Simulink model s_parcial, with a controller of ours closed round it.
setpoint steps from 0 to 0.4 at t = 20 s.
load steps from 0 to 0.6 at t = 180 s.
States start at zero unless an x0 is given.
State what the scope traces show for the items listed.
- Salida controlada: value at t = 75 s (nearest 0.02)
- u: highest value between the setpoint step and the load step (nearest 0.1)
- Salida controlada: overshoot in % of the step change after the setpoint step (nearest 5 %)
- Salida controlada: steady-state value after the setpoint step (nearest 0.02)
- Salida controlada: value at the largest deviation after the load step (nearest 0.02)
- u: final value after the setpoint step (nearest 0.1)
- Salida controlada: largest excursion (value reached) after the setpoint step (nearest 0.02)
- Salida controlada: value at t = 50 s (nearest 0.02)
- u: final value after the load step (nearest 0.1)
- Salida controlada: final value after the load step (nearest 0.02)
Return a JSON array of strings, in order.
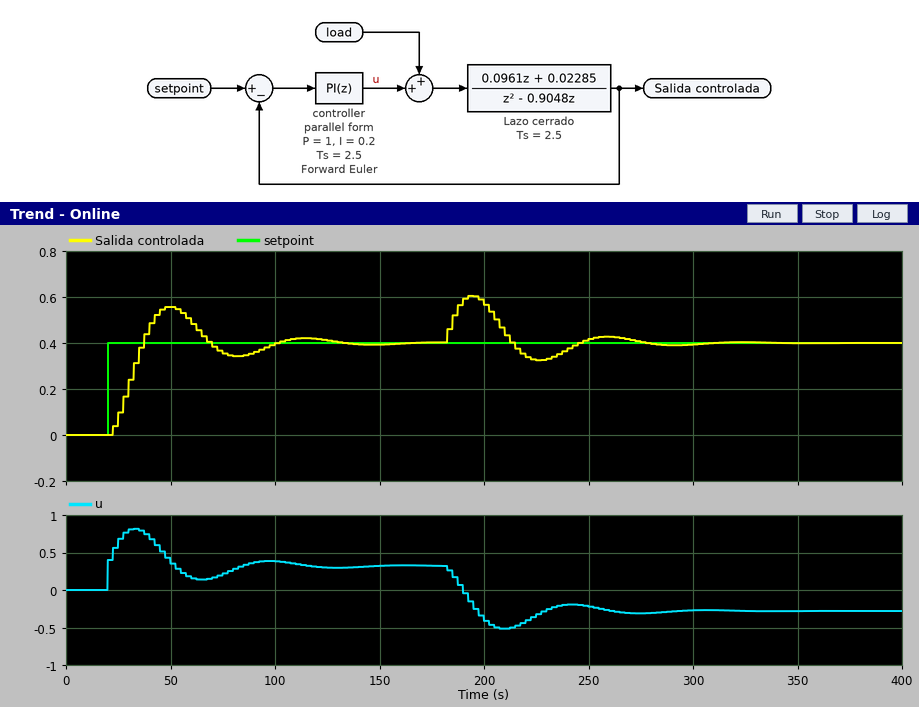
["0.36", "0.8", "40 %", "0.40", "0.60", "0.3", "0.56", "0.56", "-0.3", "0.40"]
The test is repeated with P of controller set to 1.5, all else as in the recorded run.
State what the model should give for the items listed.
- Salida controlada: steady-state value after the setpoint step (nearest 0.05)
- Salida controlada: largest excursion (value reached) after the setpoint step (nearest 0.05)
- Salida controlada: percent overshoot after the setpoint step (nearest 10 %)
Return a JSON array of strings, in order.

["0.40", "0.50", "30 %"]
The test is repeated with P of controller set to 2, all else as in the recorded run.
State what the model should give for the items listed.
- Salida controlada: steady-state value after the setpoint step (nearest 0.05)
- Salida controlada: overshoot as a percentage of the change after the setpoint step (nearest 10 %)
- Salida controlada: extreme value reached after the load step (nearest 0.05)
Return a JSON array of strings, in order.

["0.40", "20 %", "0.55"]
